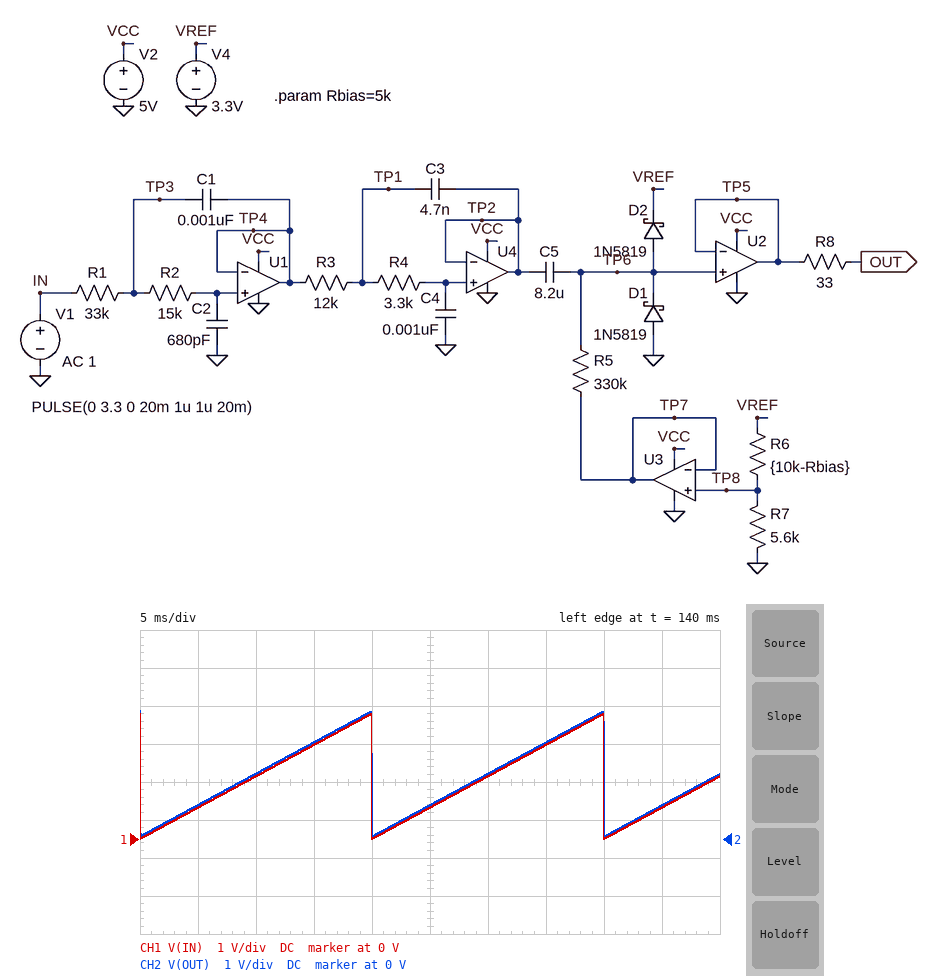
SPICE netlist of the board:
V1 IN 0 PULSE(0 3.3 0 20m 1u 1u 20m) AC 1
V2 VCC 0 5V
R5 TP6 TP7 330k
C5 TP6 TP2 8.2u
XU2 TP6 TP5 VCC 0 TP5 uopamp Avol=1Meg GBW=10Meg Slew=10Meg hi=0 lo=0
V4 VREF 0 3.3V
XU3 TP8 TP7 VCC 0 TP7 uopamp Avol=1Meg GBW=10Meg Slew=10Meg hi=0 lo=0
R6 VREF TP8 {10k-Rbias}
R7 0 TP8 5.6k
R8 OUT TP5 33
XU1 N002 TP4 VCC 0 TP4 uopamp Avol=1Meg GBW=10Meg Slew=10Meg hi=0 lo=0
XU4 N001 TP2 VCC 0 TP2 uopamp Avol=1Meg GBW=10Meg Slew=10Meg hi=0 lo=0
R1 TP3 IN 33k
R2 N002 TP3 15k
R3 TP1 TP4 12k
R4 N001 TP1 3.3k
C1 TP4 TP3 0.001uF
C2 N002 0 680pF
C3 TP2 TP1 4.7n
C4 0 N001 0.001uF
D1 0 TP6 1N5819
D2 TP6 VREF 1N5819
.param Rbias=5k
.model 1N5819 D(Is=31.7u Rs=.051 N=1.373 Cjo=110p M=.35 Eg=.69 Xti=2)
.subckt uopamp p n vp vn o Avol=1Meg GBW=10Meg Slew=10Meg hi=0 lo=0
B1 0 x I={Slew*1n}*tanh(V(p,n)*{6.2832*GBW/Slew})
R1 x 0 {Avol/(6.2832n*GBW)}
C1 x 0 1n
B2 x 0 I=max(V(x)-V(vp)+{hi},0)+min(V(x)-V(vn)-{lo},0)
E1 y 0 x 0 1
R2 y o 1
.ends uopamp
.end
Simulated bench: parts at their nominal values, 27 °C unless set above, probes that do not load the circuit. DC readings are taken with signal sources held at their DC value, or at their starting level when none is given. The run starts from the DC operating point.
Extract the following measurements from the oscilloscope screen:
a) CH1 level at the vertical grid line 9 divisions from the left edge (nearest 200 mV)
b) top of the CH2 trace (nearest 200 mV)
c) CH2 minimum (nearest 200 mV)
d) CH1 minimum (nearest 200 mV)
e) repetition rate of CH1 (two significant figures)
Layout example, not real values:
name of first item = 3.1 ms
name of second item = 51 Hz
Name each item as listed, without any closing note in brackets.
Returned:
CH1 level at the vertical grid line 9 divisions from the left edge = 800 mV
top of the CH2 trace = 3.4 V
CH2 minimum = 0 V
CH1 minimum = 0 V
repetition rate of CH1 = 50 Hz
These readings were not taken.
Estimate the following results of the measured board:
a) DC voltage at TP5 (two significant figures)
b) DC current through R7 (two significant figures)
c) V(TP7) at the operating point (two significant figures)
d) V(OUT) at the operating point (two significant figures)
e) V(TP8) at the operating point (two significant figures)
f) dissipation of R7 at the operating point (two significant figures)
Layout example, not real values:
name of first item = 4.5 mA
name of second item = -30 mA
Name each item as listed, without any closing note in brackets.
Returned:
DC voltage at TP5 = 1.7 V
DC current through R7 = 310 µA
V(TP7) at the operating point = 1.7 V
V(OUT) at the operating point = 1.7 V
V(TP8) at the operating point = 1.7 V
dissipation of R7 at the operating point = 540 µW
